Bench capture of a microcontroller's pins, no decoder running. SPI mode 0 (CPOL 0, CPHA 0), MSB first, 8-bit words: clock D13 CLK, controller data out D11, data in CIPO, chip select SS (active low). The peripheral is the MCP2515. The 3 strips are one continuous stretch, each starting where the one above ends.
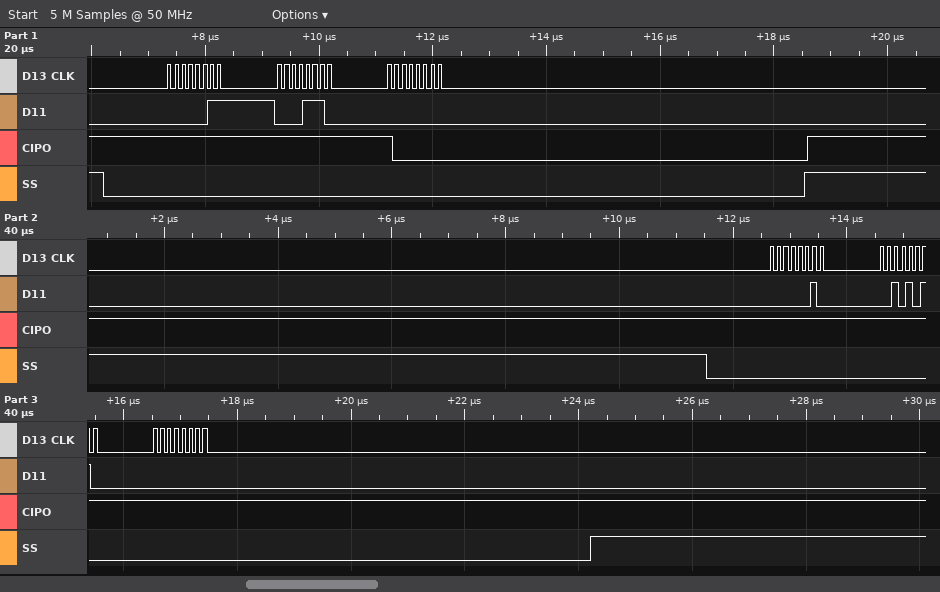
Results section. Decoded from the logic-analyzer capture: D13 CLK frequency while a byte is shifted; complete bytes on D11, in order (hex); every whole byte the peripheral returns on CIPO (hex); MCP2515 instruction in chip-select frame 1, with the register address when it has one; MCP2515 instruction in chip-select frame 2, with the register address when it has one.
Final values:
8 MHz
0x03 0x0E 0x00 0x02 0x2A 0x00
0xFF 0xFF 0x80 0xFF 0xFF 0xFF
READ 0x0E
WRITE 0x2A
